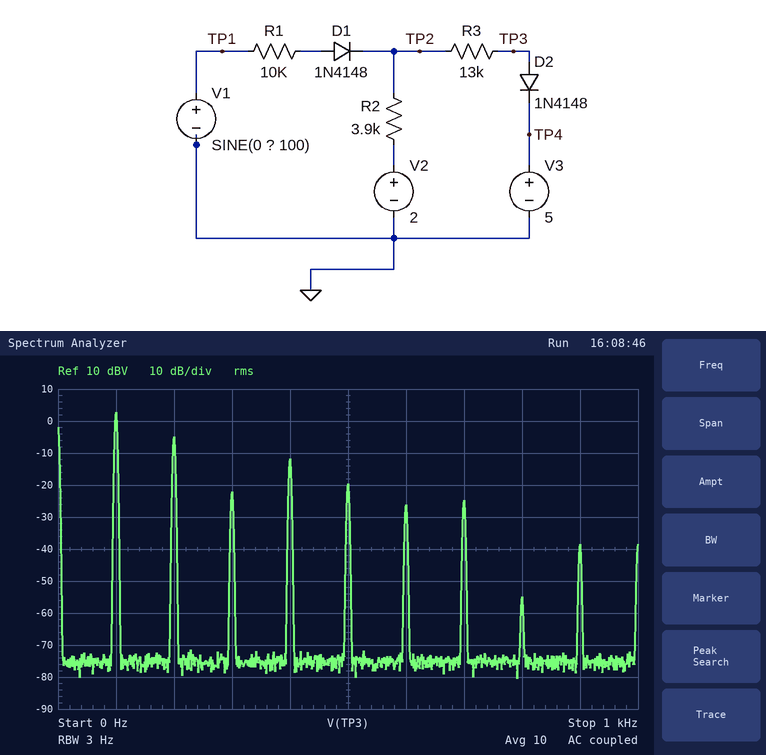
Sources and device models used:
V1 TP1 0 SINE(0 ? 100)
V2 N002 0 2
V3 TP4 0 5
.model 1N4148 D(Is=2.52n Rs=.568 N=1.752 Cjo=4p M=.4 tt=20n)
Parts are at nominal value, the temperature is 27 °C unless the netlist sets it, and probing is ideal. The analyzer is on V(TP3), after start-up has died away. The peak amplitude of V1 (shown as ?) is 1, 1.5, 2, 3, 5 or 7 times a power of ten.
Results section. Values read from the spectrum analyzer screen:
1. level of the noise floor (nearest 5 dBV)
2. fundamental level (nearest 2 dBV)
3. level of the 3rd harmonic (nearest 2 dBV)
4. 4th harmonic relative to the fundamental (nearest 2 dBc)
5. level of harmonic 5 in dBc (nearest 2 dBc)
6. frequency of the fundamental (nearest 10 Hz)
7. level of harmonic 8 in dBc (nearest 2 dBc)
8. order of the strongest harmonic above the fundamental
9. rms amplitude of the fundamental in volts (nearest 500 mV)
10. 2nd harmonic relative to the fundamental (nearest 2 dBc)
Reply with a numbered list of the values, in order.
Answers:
1. -75 dBV
2. 2 dBV
3. -22 dBV
4. -14 dBc
5. -22 dBc
6. 100 Hz
7. -58 dBc
8. 2
9. 1.5 V
10. -8 dBc
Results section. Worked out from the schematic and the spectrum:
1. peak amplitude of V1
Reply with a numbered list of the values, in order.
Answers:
1. 20 V
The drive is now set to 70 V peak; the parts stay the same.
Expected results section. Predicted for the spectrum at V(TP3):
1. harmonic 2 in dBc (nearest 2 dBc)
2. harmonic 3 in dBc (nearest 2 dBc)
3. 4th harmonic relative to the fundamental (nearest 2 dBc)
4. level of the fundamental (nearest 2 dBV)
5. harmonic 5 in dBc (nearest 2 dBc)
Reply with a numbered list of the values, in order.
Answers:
1. -18 dBc
2. -10 dBc
3. -18 dBc
4. 4 dBV
5. -16 dBc
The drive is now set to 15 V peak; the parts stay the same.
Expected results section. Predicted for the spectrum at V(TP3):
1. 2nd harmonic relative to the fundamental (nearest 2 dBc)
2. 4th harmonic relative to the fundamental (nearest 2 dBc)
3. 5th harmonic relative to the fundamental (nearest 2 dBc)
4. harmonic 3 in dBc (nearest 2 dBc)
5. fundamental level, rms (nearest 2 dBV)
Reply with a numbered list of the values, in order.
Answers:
1. -6 dBc
2. -20 dBc
3. -26 dBc
4. -22 dBc
5. 2 dBV
